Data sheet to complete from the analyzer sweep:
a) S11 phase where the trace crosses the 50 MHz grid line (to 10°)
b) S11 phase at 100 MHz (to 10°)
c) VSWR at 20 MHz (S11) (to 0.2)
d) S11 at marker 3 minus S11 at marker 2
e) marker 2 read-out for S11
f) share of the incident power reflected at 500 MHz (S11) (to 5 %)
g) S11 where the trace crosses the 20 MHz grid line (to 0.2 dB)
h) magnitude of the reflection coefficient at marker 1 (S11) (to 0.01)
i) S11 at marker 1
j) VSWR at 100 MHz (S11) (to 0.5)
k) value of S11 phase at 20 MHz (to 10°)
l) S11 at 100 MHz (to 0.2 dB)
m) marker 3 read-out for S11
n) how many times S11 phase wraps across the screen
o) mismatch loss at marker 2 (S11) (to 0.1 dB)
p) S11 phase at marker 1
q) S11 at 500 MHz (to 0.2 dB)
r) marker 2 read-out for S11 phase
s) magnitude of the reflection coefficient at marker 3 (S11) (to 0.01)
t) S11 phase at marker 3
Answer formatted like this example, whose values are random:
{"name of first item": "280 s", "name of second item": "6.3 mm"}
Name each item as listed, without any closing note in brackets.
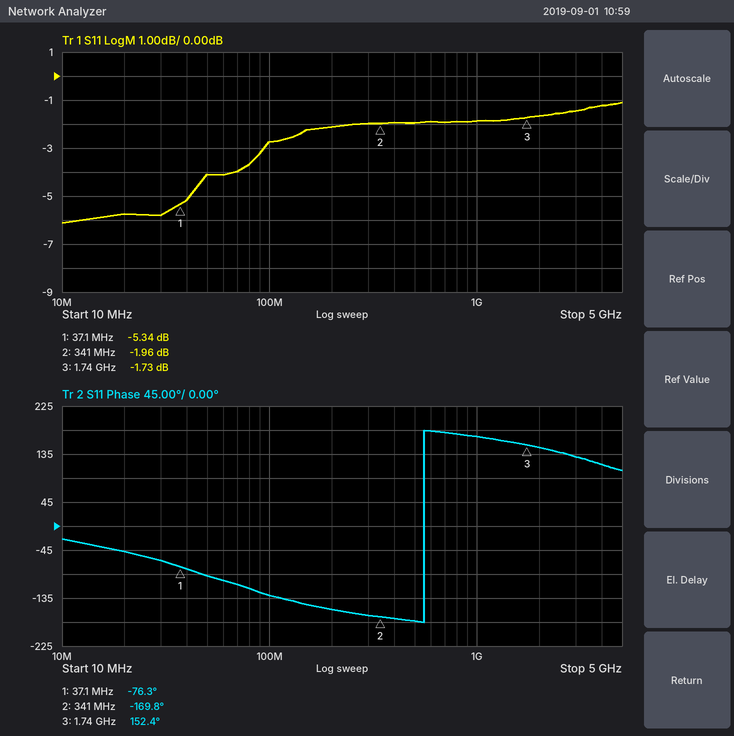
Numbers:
{"S11 phase where the trace crosses the 50 MHz grid line": "-90°", "S11 phase at 100 MHz": "-130°", "VSWR at 20 MHz (S11)": "3.2", "S11 at marker 3 minus S11 at marker 2": "0.23 dB", "marker 2 read-out for S11": "-1.96 dB", "share of the incident power reflected at 500 MHz (S11)": "65 %", "S11 where the trace crosses the 20 MHz grid line": "-5.8 dB", "magnitude of the reflection coefficient at marker 1 (S11)": "0.54", "S11 at marker 1": "-5.34 dB", "VSWR at 100 MHz (S11)": "6.5", "value of S11 phase at 20 MHz": "-50°", "S11 at 100 MHz": "-2.8 dB", "marker 3 read-out for S11": "-1.73 dB", "how many times S11 phase wraps across the screen": "1", "mismatch loss at marker 2 (S11)": "4.4 dB", "S11 phase at marker 1": "-76.3°", "S11 at 500 MHz": "-2.0 dB", "marker 2 read-out for S11 phase": "-169.8°", "magnitude of the reflection coefficient at marker 3 (S11)": "0.82", "S11 phase at marker 3": "152.4°"}
